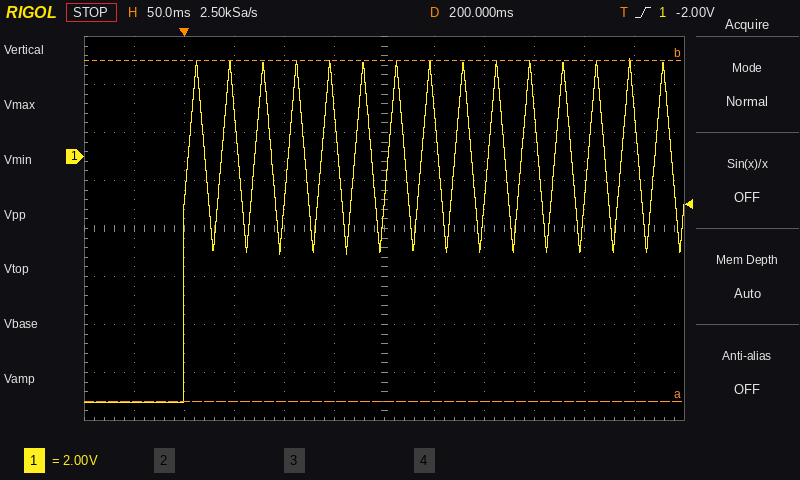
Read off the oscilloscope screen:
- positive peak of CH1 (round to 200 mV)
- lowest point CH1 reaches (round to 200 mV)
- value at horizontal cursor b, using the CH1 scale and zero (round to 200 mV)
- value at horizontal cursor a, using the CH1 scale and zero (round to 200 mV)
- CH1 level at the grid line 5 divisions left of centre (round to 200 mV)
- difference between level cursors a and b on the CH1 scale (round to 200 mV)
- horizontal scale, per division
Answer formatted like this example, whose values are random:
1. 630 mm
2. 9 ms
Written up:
1. 4.0 V
2. -10.2 V
3. 4.0 V
4. -10.2 V
5. -10.2 V
6. 14.2 V
7. 50 ms
